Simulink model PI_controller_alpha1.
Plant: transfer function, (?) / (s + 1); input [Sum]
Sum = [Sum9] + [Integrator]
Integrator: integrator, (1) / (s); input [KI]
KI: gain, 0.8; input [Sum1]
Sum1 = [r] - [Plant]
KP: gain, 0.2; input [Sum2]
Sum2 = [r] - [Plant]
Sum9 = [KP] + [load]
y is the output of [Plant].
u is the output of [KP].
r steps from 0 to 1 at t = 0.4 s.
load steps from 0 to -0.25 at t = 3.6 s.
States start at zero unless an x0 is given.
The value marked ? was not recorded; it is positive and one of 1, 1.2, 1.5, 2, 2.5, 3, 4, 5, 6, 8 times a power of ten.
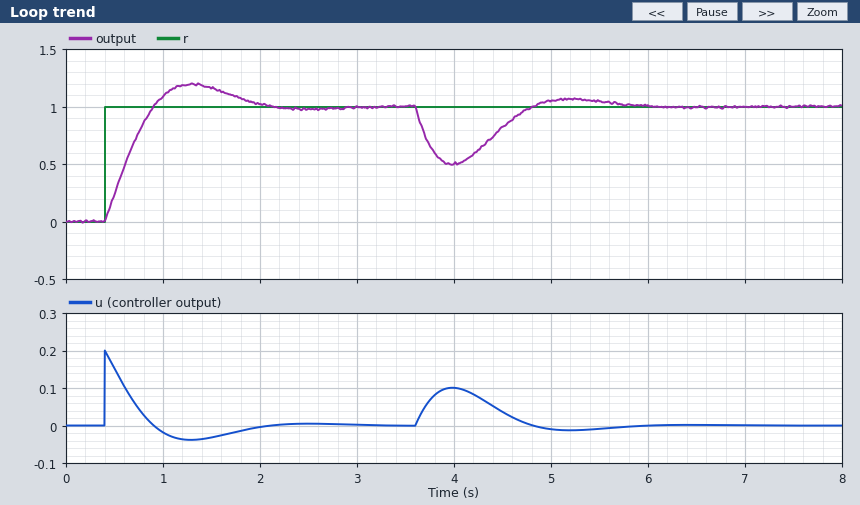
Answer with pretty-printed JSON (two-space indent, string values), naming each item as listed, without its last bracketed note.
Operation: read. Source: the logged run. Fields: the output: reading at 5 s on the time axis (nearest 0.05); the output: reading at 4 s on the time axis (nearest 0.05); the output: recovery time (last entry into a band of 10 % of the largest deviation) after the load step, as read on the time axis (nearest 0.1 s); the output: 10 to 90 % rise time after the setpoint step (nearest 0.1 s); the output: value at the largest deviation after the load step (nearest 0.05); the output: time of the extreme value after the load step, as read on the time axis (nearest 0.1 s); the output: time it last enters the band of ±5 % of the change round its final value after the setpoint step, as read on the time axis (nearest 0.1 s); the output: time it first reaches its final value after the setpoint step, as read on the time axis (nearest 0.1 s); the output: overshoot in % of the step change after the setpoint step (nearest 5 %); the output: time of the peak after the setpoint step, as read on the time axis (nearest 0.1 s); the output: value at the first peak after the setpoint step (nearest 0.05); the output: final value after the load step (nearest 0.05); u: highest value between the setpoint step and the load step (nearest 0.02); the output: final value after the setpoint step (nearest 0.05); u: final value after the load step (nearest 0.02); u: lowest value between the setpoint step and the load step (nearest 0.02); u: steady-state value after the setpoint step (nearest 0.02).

{
  "the output: reading at 5 s on the time axis": "1.05",
  "the output: reading at 4 s on the time axis": "0.50",
  "the output: recovery time (last entry into a band of 10 % of the largest deviation) after the load step, as read on the time axis": "5.4 s",
  "the output: 10 to 90 % rise time after the setpoint step": "0.4 s",
  "the output: value at the largest deviation after the load step": "0.50",
  "the output: time of the extreme value after the load step, as read on the time axis": "4.0 s",
  "the output: time it last enters the band of ±5 % of the change round its final value after the setpoint step, as read on the time axis": "1.9 s",
  "the output: time it first reaches its final value after the setpoint step, as read on the time axis": "0.9 s",
  "the output: overshoot in % of the step change after the setpoint step": "20 %",
  "the output: time of the peak after the setpoint step, as read on the time axis": "1.3 s",
  "the output: value at the first peak after the setpoint step": "1.20",
  "the output: final value after the load step": "1.00",
  "u: highest value between the setpoint step and the load step": "0.20",
  "the output: final value after the setpoint step": "1.00",
  "u: final value after the load step": "0.00",
  "u: lowest value between the setpoint step and the load step": "-0.04",
  "u: steady-state value after the setpoint step": "0.00"
}
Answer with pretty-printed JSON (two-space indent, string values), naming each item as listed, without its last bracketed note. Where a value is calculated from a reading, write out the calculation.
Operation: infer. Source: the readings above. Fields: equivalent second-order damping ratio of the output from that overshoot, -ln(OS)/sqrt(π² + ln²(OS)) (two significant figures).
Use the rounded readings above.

{
  "equivalent second-order damping ratio of the output from that overshoot, -ln(OS)/sqrt(π² + ln²(OS))": "ln(0.2) = -1.609; 1.609 / sqrt(9.870 + 2.590) = 0.46"
}
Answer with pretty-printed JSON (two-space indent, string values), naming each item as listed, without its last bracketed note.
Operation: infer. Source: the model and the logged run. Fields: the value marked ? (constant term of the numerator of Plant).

{
  "the value marked ?": "12"
}
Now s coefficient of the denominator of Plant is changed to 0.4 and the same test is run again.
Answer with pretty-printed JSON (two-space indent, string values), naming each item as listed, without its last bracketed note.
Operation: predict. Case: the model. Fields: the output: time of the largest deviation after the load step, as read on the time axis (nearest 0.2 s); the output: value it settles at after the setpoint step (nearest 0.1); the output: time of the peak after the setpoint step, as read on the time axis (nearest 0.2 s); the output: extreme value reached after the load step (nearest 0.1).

{
  "the output: time of the largest deviation after the load step, as read on the time axis": "3.8 s",
  "the output: value it settles at after the setpoint step": "1.0",
  "the output: time of the peak after the setpoint step, as read on the time axis": "1.0 s",
  "the output: extreme value reached after the load step": "0.4"
}
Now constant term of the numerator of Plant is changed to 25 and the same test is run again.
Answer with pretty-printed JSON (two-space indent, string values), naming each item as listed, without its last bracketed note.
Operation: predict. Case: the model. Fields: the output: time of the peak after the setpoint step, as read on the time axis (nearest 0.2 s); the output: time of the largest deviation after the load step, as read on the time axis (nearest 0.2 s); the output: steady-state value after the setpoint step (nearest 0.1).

{
  "the output: time of the peak after the setpoint step, as read on the time axis": "1.0 s",
  "the output: time of the largest deviation after the load step, as read on the time axis": "3.8 s",
  "the output: steady-state value after the setpoint step": "1.0"
}
